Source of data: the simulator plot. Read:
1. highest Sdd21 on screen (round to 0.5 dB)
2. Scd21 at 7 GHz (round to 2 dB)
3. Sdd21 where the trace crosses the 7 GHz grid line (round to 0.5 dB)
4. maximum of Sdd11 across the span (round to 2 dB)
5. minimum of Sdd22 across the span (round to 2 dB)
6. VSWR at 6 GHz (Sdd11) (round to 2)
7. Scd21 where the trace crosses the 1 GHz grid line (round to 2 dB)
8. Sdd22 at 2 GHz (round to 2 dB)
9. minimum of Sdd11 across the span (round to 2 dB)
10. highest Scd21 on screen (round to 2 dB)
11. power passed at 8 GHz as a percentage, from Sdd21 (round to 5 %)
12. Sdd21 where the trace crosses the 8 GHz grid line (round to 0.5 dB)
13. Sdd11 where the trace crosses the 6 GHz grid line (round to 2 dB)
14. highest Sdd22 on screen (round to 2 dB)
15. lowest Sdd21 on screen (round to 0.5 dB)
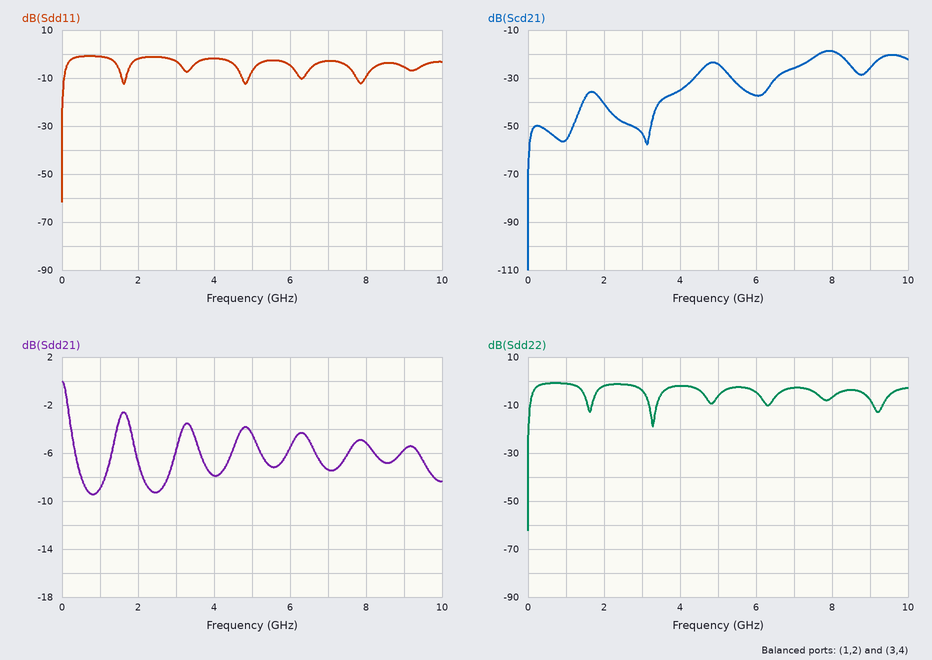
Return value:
0.0 dB
-26 dB
-7.5 dB
0 dB
-62 dB
4
-56 dB
-2 dB
-62 dB
-18 dB
30 %
-5.0 dB
-4 dB
0 dB
-9.5 dB
